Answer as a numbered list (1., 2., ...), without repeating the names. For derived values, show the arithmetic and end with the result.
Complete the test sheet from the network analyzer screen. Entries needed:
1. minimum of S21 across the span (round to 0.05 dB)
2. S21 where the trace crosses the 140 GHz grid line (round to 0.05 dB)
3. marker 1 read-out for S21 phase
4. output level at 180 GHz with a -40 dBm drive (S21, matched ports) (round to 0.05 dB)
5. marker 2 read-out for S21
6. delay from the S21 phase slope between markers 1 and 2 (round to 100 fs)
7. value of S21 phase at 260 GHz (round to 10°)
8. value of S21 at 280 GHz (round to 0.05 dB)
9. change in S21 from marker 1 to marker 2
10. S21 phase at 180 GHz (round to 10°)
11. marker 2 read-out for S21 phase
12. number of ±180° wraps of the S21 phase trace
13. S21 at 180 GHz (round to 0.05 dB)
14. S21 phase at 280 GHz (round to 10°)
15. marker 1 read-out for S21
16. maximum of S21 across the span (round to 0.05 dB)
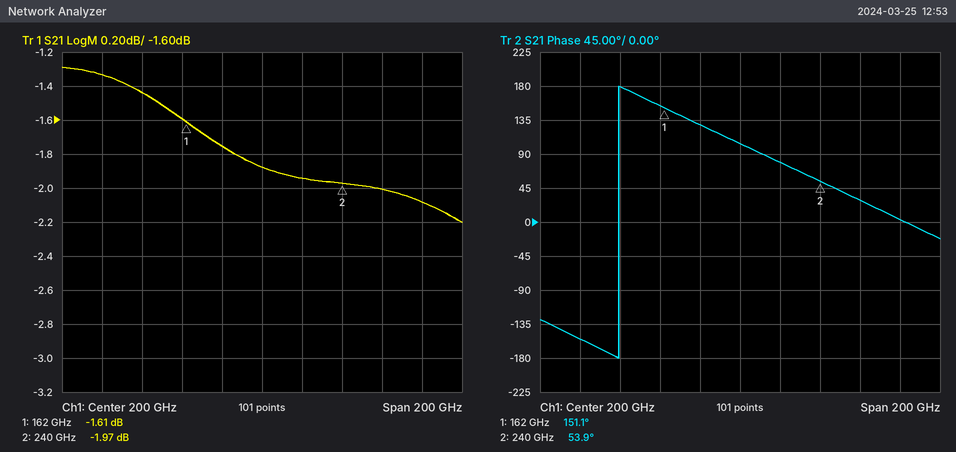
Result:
1. -2.20 dB
2. -1.45 dB
3. 151.1°
4. -40 dBm + (-1.75 dB) = -41.75 dBm
5. -1.97 dB
6. −(53.9° − (151.1°))/(360° × 78 GHz) ≈ 3.5 ps
7. 30°
8. -2.10 dB
9. -1.97 − (-1.61) = -0.36 dB
10. 130°
11. 53.9°
12. 1
13. -1.75 dB
14. 0°
15. -1.61 dB
16. -1.30 dB
